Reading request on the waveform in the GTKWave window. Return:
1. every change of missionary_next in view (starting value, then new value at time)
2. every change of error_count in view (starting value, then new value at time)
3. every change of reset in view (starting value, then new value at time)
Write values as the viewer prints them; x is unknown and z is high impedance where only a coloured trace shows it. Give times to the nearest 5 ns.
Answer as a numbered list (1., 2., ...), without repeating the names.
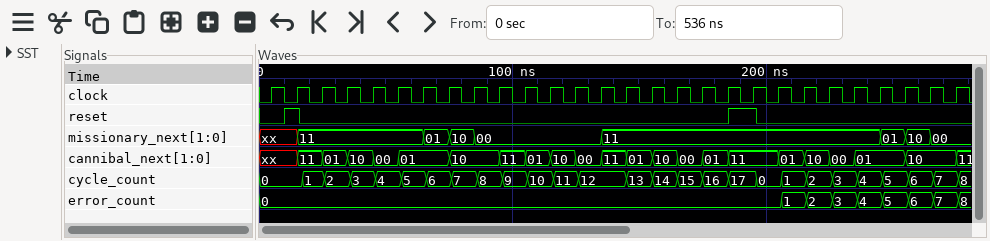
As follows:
1. xx, 11 at 15 ns, 01 at 65 ns, 10 at 75 ns, 00 at 85 ns, 11 at 135 ns, 01 at 245 ns, 10 at 255 ns, 00 at 265 ns
2. 0, 1 at 205 ns, 2 at 215 ns, 3 at 225 ns, 4 at 235 ns, 5 at 245 ns, 6 at 255 ns, 7 at 265 ns, 8 at 275 ns
3. 0, 1 at 10 ns, 0 at 15 ns, 1 at 185 ns, 0 at 195 ns
